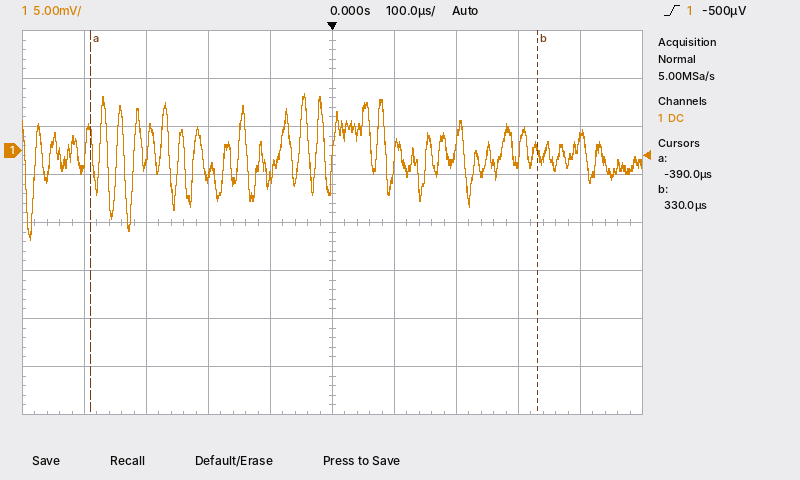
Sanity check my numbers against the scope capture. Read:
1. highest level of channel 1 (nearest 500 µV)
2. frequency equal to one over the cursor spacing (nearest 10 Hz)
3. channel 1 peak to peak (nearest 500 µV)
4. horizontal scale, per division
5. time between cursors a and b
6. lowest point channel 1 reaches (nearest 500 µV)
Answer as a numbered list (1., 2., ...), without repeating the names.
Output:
1. 6.0 mV
2. 1.39 kHz
3. 15.5 mV
4. 100 µs
5. 720 µs
6. -9.5 mV
